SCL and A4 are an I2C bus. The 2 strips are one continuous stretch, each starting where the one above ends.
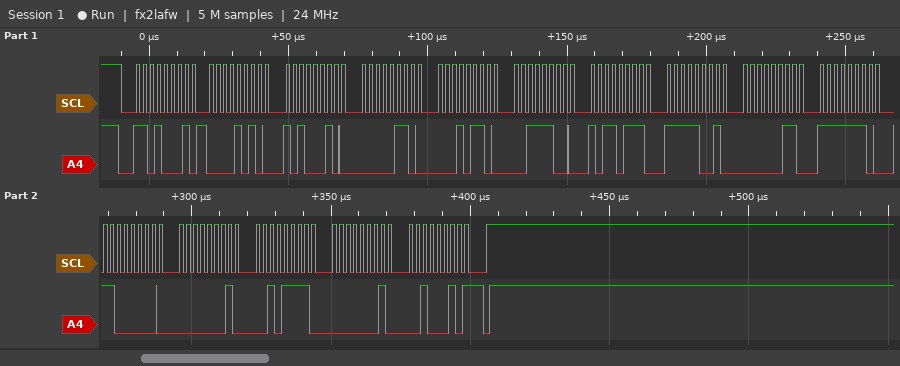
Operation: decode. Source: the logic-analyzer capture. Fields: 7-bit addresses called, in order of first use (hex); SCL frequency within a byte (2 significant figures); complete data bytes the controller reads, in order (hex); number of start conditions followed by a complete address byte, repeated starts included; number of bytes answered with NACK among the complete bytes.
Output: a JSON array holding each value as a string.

["0x68", "400 kHz", "0A A2 06 16 3C B7 F9 03 FE C0 01 2F 01 22", "1", "1"]
